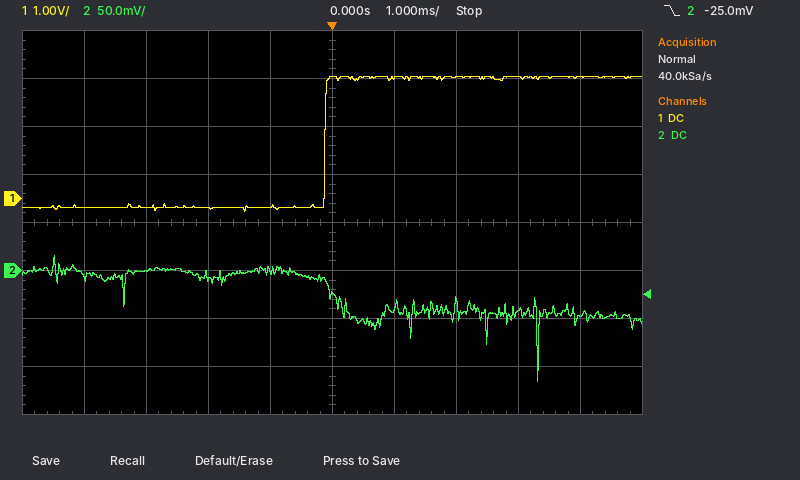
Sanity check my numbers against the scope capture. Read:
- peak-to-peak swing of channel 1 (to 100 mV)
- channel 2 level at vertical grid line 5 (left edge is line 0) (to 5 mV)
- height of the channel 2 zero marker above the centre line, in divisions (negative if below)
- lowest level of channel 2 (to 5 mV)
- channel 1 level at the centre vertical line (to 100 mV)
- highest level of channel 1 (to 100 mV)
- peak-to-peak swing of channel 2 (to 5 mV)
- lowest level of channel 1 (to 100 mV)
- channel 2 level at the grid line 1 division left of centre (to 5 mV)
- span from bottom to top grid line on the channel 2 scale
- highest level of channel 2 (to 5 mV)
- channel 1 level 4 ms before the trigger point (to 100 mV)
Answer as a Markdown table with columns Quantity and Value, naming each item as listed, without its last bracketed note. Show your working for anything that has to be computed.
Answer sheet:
| Quantity | Value |
|---|---|
| peak-to-peak swing of channel 1 | 2.5 V − (-300 mV) = 2.8 V |
| channel 2 level at vertical grid line 5 (left edge is line 0) | -25 mV |
| height of the channel 2 zero marker above the centre line, in divisions | -1.0 div |
| lowest level of channel 2 | -115 mV |
| channel 1 level at the centre vertical line | 2.5 V |
| highest level of channel 1 | 2.5 V |
| peak-to-peak swing of channel 2 | 15 mV − (-115 mV) = 130 mV |
| lowest level of channel 1 | -300 mV |
| channel 2 level at the grid line 1 division left of centre | 0 mV |
| span from bottom to top grid line on the channel 2 scale | 400 mV |
| highest level of channel 2 | 15 mV |
| channel 1 level 4 ms before the trigger point | -200 mV |
